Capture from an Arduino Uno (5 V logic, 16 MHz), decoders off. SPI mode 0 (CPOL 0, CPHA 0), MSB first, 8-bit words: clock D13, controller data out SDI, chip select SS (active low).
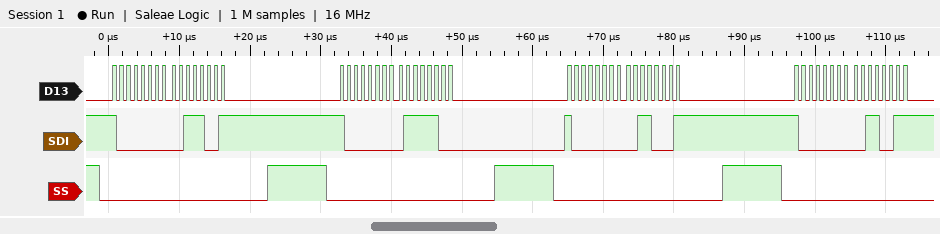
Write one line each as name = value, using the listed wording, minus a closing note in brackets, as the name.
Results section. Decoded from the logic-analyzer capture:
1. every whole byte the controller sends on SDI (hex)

every whole byte the controller sends on SDI = 0x80 0x39 0x80 0x7C 0x80 0x31 0x80 0x33
